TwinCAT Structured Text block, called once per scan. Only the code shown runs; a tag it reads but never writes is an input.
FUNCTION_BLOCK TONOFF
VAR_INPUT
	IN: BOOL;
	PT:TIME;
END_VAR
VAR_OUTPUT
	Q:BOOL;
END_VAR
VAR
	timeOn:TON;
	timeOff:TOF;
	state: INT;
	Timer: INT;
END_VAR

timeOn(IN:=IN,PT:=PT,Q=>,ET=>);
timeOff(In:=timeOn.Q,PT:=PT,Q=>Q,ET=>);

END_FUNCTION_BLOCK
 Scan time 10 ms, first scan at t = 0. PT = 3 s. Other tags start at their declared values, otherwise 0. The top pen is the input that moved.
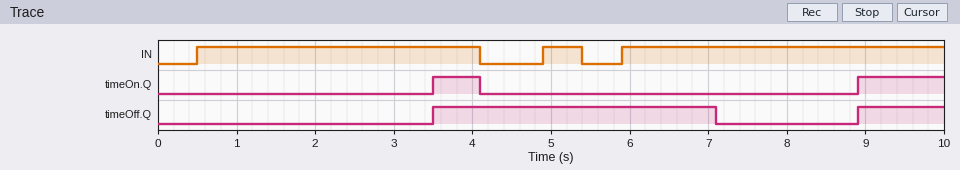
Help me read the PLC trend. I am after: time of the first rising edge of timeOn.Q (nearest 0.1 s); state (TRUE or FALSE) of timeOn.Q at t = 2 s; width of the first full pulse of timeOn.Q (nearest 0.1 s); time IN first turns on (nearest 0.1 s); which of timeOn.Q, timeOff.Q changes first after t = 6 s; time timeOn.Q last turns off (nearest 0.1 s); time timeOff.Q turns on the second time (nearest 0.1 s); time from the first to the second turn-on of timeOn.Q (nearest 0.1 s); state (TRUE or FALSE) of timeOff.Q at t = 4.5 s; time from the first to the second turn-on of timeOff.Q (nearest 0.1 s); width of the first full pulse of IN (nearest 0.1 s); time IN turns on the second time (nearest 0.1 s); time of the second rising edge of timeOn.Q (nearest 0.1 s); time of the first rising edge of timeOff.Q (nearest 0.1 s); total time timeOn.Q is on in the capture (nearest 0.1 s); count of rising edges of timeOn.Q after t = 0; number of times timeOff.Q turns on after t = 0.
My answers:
3.5 s
FALSE
0.6 s
0.5 s
timeOff.Q
4.1 s
8.9 s
5.4 s
TRUE
5.4 s
3.6 s
4.9 s
8.9 s
3.5 s
1.7 s
2
2
